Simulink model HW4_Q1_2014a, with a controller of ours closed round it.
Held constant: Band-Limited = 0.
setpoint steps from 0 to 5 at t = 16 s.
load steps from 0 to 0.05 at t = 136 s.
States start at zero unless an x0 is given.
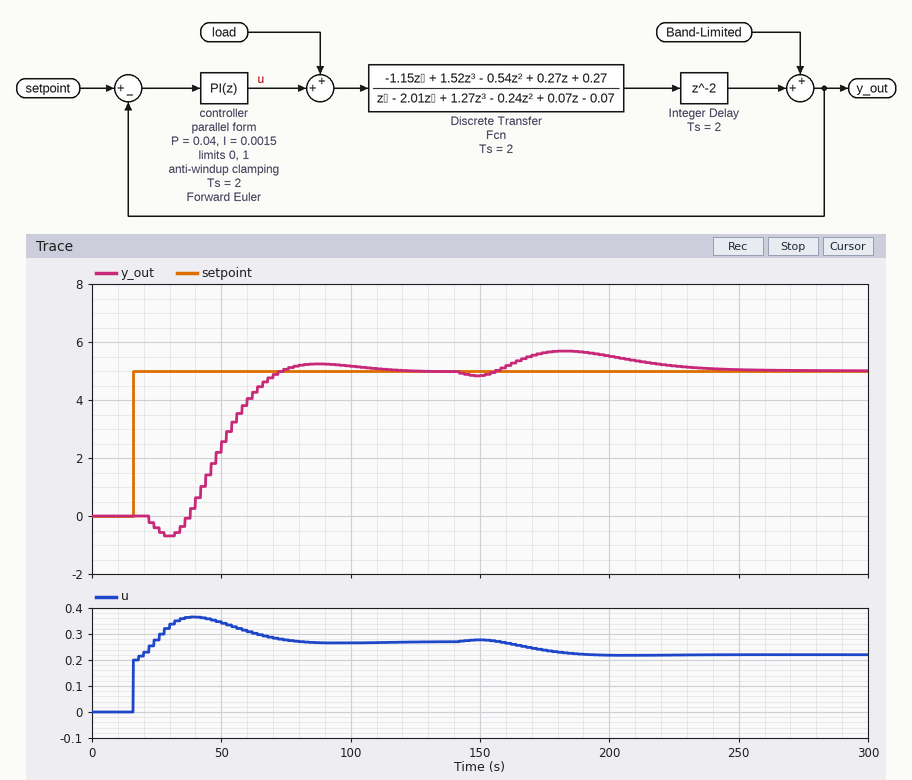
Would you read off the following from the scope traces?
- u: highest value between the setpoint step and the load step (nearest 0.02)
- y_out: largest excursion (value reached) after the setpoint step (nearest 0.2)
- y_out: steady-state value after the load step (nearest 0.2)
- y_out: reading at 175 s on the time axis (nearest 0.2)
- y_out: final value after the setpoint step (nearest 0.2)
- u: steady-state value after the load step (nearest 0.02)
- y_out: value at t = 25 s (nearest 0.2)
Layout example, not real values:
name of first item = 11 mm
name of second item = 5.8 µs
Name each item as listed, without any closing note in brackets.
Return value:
u: highest value between the setpoint step and the load step = 0.36
y_out: largest excursion (value reached) after the setpoint step = 5.2
y_out: steady-state value after the load step = 5.0
y_out: reading at 175 s on the time axis = 5.6
y_out: final value after the setpoint step = 5.0
u: steady-state value after the load step = 0.22
y_out: value at t = 25 s = -0.4
